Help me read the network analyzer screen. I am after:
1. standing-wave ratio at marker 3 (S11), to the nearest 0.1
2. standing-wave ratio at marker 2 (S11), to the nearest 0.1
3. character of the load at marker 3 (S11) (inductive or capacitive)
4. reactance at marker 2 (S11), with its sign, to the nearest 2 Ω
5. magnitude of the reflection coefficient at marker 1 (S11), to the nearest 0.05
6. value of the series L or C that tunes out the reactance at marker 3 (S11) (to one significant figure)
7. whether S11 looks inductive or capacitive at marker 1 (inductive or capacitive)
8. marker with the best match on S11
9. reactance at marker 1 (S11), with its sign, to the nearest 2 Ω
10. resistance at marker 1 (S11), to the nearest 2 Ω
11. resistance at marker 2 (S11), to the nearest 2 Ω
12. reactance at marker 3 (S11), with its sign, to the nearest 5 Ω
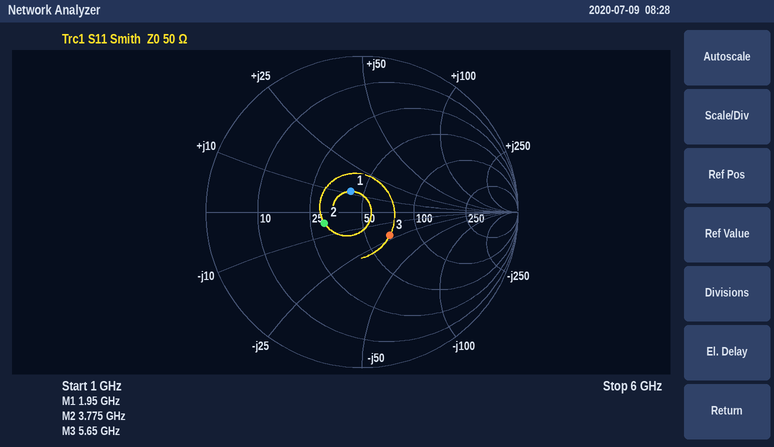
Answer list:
1.6
1.7
capacitive
-4 Ω
0.15
600 pH
inductive
marker 1
+12 Ω
42 Ω
30 Ω
-20 Ω
